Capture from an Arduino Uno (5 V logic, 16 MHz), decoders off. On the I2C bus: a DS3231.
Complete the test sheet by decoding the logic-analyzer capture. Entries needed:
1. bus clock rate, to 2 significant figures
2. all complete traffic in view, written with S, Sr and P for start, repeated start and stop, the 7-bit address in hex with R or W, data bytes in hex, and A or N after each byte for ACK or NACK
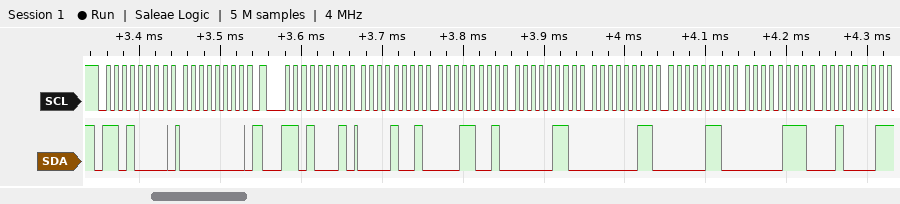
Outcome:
100 kHz
S 68W A 00 A Sr 68R A 09 A 19 A 06 A 03 A 06 A 07 A 21 N
